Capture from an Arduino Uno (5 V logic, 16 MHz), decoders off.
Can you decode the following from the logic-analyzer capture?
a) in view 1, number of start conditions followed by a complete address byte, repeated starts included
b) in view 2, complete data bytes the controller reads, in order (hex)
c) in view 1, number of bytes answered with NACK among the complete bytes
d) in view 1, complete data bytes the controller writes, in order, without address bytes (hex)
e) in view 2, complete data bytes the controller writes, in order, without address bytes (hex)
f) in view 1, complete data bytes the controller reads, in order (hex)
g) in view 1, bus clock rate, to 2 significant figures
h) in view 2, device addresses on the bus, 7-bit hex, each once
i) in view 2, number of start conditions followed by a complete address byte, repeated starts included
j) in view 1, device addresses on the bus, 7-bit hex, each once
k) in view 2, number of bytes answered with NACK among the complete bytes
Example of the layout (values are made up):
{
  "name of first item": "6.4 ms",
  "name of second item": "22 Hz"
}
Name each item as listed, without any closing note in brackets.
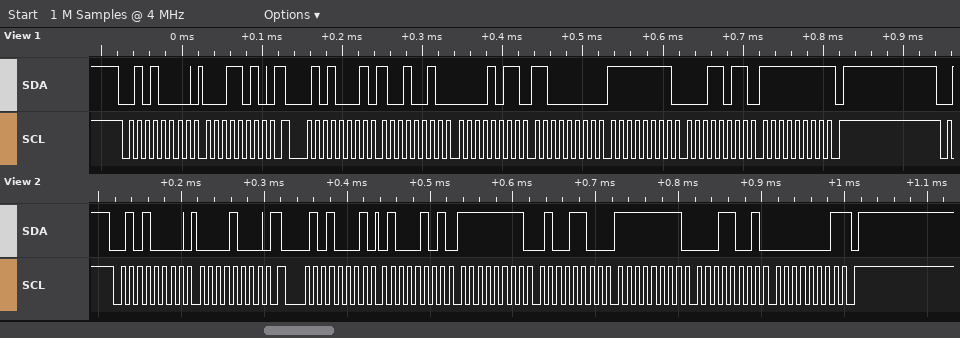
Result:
{
  "in view 1, number of start conditions followed by a complete address byte, repeated starts included": "2",
  "in view 2, complete data bytes the controller reads, in order": "45 FF 4C FF 19 01",
  "in view 1, number of bytes answered with NACK among the complete bytes": "1",
  "in view 1, complete data bytes the controller writes, in order, without address bytes": "1A",
  "in view 2, complete data bytes the controller writes, in order, without address bytes": "08",
  "in view 1, complete data bytes the controller reads, in order": "92 0B C0 FF 1B FF",
  "in view 1, bus clock rate, to 2 significant figures": "100 kHz",
  "in view 2, device addresses on the bus, 7-bit hex, each once": "0x28",
  "in view 2, number of start conditions followed by a complete address byte, repeated starts included": "2",
  "in view 1, device addresses on the bus, 7-bit hex, each once": "0x28",
  "in view 2, number of bytes answered with NACK among the complete bytes": "1"
}
